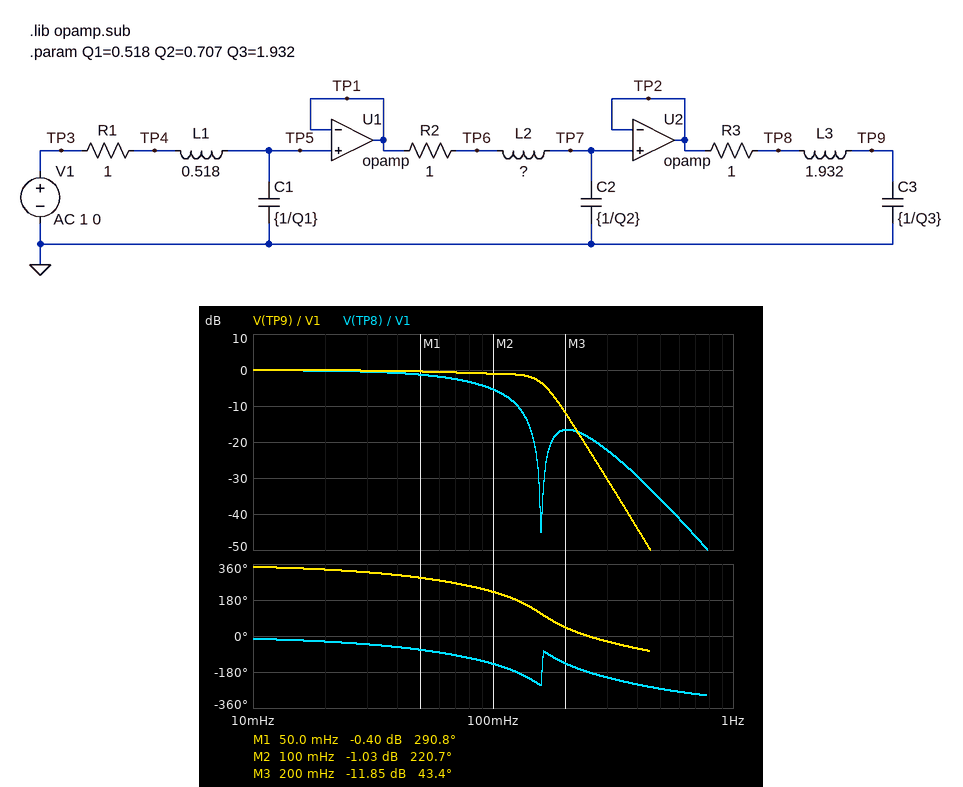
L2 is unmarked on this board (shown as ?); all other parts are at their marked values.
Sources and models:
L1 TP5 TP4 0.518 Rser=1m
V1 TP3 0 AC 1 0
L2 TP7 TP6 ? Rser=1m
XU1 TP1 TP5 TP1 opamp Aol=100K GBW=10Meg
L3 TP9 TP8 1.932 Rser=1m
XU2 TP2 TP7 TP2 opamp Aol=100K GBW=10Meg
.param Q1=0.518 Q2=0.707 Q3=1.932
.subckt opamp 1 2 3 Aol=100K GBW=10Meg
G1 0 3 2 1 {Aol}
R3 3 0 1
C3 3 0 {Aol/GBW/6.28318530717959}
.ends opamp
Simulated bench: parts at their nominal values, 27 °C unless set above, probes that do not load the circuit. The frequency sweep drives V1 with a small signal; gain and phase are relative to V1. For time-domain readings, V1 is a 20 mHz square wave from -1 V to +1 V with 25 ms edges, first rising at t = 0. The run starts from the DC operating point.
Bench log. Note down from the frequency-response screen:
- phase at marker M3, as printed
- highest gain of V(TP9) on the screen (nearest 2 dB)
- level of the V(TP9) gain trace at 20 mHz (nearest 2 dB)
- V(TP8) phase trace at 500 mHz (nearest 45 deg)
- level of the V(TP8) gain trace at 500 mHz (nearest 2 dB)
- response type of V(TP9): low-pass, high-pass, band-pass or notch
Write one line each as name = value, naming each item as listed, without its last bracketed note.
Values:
phase at marker M3, as printed = 43.4 deg
highest gain of V(TP9) on the screen = 0 dB
level of the V(TP9) gain trace at 20 mHz = 0 dB
V(TP8) phase trace at 500 mHz = -270 deg
level of the V(TP8) gain trace at 500 mHz = -36 dB
response type of V(TP9): low-pass, high-pass, band-pass or notch = low-pass
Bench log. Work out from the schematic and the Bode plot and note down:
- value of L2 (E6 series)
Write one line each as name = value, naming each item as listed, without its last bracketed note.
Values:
value of L2 = 330 mH
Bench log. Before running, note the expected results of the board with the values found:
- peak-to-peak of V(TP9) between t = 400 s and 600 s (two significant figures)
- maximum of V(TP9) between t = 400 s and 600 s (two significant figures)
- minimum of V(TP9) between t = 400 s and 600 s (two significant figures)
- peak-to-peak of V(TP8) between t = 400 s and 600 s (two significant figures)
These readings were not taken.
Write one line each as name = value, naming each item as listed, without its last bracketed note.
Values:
peak-to-peak of V(TP9) between t = 400 s and 600 s = 2.3 V
maximum of V(TP9) between t = 400 s and 600 s = 1.2 V
minimum of V(TP9) between t = 400 s and 600 s = -1.2 V
peak-to-peak of V(TP8) between t = 400 s and 600 s = 2.1 V
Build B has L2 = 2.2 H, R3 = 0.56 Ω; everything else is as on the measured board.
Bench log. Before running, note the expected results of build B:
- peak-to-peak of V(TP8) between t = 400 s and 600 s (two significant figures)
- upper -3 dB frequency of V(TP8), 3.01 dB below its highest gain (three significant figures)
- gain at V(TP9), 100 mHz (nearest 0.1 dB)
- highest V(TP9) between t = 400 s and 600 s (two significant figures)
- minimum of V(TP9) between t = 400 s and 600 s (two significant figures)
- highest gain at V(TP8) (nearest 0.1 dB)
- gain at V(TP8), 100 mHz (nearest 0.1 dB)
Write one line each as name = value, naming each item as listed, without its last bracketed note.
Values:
peak-to-peak of V(TP8) between t = 400 s and 600 s = 2.8 V
upper -3 dB frequency of V(TP8), 3.01 dB below its highest gain = 97.6 mHz
gain at V(TP9), 100 mHz = 2.1 dB
highest V(TP9) between t = 400 s and 600 s = 1.7 V
minimum of V(TP9) between t = 400 s and 600 s = -1.7 V
highest gain at V(TP8) = 1.2 dB
gain at V(TP8), 100 mHz = -2.3 dB
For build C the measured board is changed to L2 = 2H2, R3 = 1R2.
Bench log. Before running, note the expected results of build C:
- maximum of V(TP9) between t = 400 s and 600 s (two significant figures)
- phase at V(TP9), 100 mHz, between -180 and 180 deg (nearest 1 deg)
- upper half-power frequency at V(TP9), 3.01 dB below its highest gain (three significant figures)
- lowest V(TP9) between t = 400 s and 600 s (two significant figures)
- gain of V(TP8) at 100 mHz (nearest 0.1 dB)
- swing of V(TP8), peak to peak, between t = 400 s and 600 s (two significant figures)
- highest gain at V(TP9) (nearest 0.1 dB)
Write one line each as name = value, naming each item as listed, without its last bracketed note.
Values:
maximum of V(TP9) between t = 400 s and 600 s = 1.6 V
phase at V(TP9), 100 mHz, between -180 and 180 deg = 159 deg
upper half-power frequency at V(TP9), 3.01 dB below its highest gain = 109 mHz
lowest V(TP9) between t = 400 s and 600 s = -1.6 V
gain of V(TP8) at 100 mHz = -3.4 dB
swing of V(TP8), peak to peak, between t = 400 s and 600 s = 2.8 V
highest gain at V(TP9) = 2.7 dB
